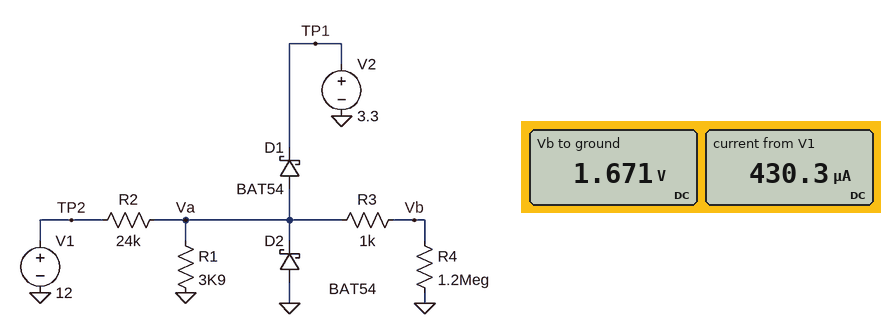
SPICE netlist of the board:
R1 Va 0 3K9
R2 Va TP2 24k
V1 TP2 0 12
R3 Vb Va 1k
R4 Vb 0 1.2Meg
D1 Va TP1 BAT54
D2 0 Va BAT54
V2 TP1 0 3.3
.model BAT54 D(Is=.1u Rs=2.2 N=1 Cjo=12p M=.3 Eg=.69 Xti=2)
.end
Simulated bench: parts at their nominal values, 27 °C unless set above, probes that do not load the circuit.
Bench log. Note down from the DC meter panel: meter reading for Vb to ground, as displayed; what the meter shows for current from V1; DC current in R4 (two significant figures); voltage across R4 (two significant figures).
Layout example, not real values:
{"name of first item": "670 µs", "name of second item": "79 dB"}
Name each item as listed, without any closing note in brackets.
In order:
{"meter reading for Vb to ground, as displayed": "1.671 V", "what the meter shows for current from V1": "430.3 µA", "DC current in R4": "1.4 µA", "voltage across R4": "1.7 V"}
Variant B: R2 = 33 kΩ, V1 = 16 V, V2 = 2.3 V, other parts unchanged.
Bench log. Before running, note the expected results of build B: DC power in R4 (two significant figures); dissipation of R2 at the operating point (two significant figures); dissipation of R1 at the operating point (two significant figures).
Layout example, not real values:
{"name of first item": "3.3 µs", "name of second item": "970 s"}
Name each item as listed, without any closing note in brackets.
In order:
{"DC power in R4": "2.4 µW", "dissipation of R2 at the operating point": "6.2 mW", "dissipation of R1 at the operating point": "730 µW"}
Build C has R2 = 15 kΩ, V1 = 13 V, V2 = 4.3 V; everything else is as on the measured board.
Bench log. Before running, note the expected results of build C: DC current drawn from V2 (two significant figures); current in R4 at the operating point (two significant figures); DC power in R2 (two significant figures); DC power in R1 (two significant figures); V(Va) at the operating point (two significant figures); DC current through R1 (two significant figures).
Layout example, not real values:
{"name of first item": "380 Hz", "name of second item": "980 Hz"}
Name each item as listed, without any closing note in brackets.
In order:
{"DC current drawn from V2": "100 nA", "current in R4 at the operating point": "2.2 µA", "DC power in R2": "7.1 mW", "DC power in R1": "1.8 mW", "V(Va) at the operating point": "2.7 V", "DC current through R1": "690 µA"}
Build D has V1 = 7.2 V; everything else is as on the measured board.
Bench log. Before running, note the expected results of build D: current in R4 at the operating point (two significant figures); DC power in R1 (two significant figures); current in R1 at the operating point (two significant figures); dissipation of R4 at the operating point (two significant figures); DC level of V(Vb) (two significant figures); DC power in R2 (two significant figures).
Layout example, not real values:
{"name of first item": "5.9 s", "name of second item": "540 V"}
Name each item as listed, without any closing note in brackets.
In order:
{"current in R4 at the operating point": "840 nA", "DC power in R1": "260 µW", "current in R1 at the operating point": "260 µA", "dissipation of R4 at the operating point": "840 nW", "DC level of V(Vb)": "1.0 V", "DC power in R2": "1.6 mW"}
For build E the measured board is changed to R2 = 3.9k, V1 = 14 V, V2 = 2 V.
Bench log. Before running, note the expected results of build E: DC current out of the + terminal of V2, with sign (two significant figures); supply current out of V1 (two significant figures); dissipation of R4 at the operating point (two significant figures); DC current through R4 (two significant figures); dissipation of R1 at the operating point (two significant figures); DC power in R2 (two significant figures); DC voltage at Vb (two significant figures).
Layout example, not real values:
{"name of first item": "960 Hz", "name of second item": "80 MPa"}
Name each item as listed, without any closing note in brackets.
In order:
{"DC current out of the + terminal of V2, with sign": "-2.4 mA", "supply current out of V1": "3.0 mA", "dissipation of R4 at the operating point": "4.3 µW", "DC current through R4": "1.9 µA", "dissipation of R1 at the operating point": "1.3 mW", "DC power in R2": "35 mW", "DC voltage at Vb": "2.3 V"}
